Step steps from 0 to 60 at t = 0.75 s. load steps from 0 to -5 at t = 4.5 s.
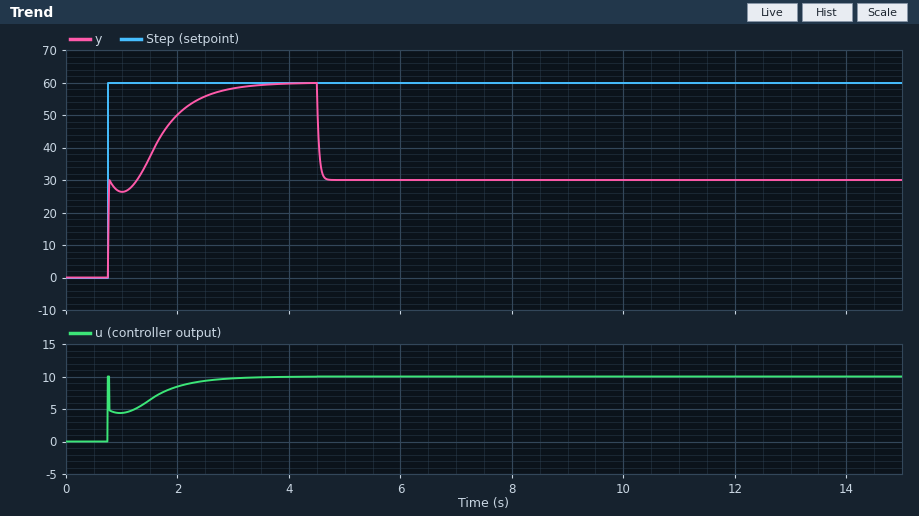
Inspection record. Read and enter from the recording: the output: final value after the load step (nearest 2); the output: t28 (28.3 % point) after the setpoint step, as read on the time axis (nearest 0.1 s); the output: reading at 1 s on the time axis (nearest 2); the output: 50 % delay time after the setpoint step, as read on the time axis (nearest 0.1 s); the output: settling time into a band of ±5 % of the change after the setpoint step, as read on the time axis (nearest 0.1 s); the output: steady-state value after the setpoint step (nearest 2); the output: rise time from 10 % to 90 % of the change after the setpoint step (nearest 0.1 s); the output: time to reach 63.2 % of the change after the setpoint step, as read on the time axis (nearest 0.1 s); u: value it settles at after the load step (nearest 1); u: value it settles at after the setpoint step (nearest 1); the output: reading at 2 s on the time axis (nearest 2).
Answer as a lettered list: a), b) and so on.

a) 30
b) 0.8 s
c) 26
d) 1.3 s
e) 2.7 s
f) 60
g) 1.5 s
h) 1.5 s
i) 10
j) 10
k) 50
